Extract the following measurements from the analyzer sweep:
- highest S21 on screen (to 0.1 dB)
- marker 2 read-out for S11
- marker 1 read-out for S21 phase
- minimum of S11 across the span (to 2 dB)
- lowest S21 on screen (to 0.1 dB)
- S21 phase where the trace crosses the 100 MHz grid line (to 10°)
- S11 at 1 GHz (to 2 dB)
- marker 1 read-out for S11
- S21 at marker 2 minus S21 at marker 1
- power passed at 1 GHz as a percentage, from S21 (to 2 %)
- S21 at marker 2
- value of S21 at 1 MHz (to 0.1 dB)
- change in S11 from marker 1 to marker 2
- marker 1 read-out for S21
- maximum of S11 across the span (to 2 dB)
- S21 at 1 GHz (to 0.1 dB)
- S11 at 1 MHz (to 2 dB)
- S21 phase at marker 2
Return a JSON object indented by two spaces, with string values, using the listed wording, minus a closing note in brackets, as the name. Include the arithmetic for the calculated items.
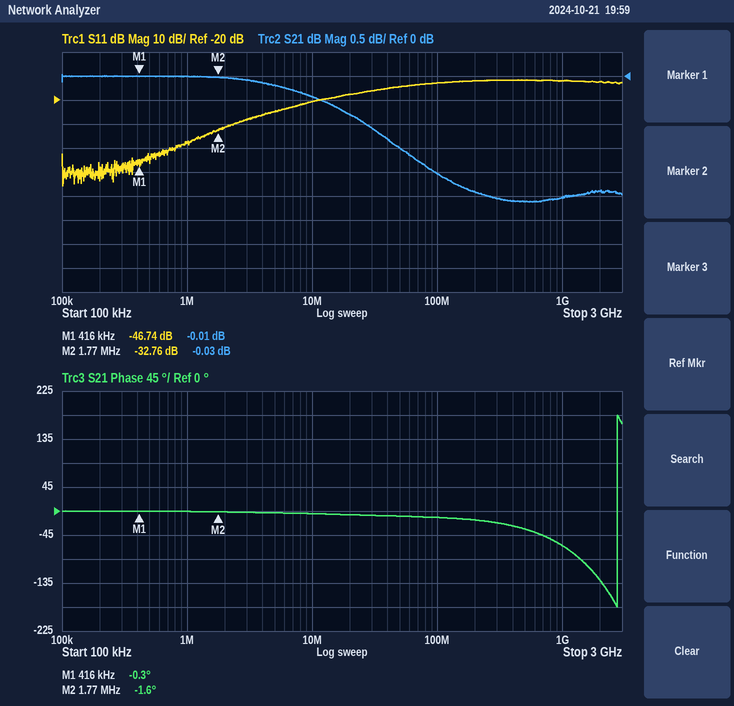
{
  "highest S21 on screen": "0.0 dB",
  "marker 2 read-out for S11": "-32.76 dB",
  "marker 1 read-out for S21 phase": "-0.3°",
  "minimum of S11 across the span": "-56 dB",
  "lowest S21 on screen": "-2.6 dB",
  "S21 phase where the trace crosses the 100 MHz grid line": "-10°",
  "S11 at 1 GHz": "-12 dB",
  "marker 1 read-out for S11": "-46.74 dB",
  "S21 at marker 2 minus S21 at marker 1": "-0.03 − (-0.01) = -0.02 dB",
  "power passed at 1 GHz as a percentage, from S21": "10^(-2.5/10) ≈ 56 %",
  "S21 at marker 2": "-0.03 dB",
  "value of S21 at 1 MHz": "0.0 dB",
  "change in S11 from marker 1 to marker 2": "-32.76 − (-46.74) = 13.98 dB",
  "marker 1 read-out for S21": "-0.01 dB",
  "maximum of S11 across the span": "-12 dB",
  "S21 at 1 GHz": "-2.5 dB",
  "S11 at 1 MHz": "-38 dB",
  "S21 phase at marker 2": "-1.6°"
}
